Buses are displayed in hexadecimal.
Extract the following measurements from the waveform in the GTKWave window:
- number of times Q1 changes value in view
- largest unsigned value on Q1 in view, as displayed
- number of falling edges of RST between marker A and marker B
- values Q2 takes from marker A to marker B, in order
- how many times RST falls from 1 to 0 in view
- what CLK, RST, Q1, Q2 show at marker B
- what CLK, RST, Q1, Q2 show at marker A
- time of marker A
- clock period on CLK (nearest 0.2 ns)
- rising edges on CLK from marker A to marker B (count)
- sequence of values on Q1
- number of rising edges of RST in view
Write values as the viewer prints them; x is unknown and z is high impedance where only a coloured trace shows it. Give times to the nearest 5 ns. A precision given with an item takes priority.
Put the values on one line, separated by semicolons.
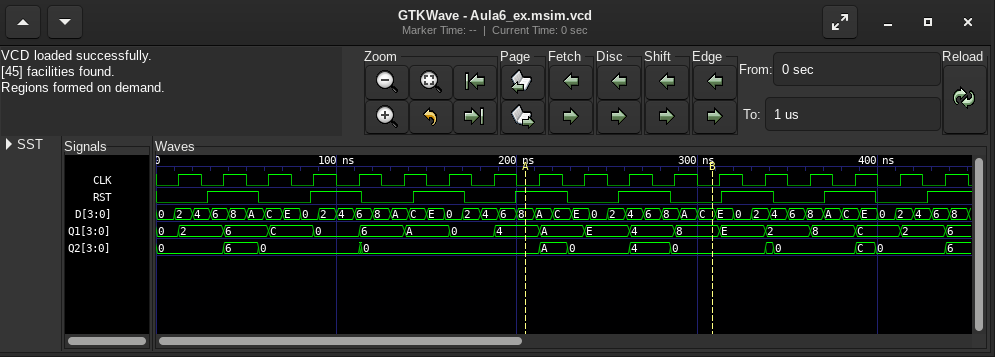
18; E; 2; 0, A, 0, 4, 0; 7; CLK=0, RST=0, Q1=8, Q2=0; CLK=0, RST=1, Q1=4, Q2=0; 205 ns; 25 ns; 4; 0, 2, 6, C, 0, 6, A, 0, 4, A, E, 4, 8, E, 2, 8, C, 2, 6; 8
